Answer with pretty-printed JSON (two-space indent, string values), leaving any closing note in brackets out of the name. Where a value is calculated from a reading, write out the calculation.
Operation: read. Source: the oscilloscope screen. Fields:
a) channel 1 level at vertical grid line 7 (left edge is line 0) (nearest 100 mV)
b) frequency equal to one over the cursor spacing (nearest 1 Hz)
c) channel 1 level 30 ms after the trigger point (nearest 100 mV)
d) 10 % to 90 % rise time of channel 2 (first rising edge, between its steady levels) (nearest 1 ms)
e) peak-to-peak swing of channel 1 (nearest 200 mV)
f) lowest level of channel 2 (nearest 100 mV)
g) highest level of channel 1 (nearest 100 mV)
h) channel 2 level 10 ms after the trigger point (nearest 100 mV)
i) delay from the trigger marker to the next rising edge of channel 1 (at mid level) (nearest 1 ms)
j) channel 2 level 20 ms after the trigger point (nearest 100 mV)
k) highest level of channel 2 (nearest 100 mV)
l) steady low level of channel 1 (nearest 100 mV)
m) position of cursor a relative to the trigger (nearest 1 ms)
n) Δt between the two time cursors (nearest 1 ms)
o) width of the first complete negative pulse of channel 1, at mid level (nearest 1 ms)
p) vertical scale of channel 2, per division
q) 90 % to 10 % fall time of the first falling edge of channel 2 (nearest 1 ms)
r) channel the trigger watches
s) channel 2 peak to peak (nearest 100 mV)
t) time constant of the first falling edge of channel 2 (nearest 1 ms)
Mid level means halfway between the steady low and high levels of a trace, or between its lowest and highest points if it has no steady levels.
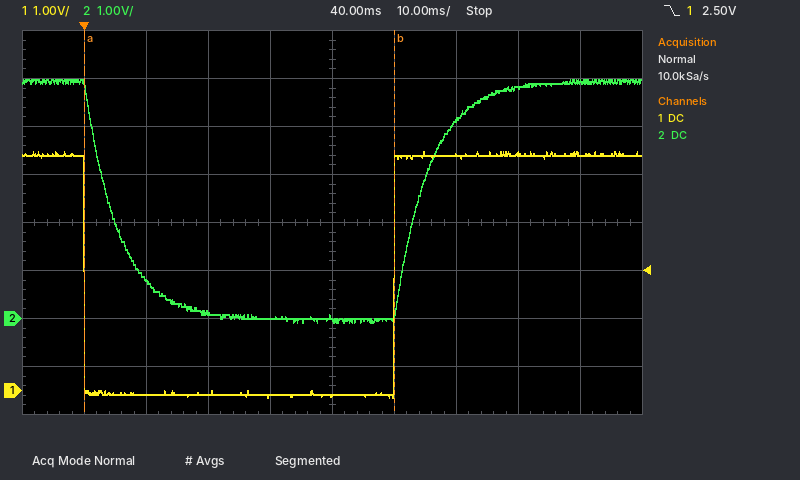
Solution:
{
  "channel 1 level at vertical grid line 7 (left edge is line 0)": "4.9 V",
  "frequency equal to one over the cursor spacing": "1 / 50 ms ≈ 20 Hz",
  "channel 1 level 30 ms after the trigger point": "-100 mV",
  "10 % to 90 % rise time of channel 2 (first rising edge, between its steady levels)": "12 ms",
  "peak-to-peak swing of channel 1": "5.2 V",
  "lowest level of channel 2": "-100 mV",
  "highest level of channel 1": "5.0 V",
  "channel 2 level 10 ms after the trigger point": "800 mV",
  "delay from the trigger marker to the next rising edge of channel 1 (at mid level)": "50 ms",
  "channel 2 level 20 ms after the trigger point": "100 mV",
  "highest level of channel 2": "5.0 V",
  "steady low level of channel 1": "-100 mV",
  "position of cursor a relative to the trigger": "0 ms",
  "Δt between the two time cursors": "50 ms",
  "width of the first complete negative pulse of channel 1, at mid level": "50 ms",
  "vertical scale of channel 2, per division": "1 V",
  "90 % to 10 % fall time of the first falling edge of channel 2": "12 ms",
  "channel the trigger watches": "channel 1",
  "channel 2 peak to peak": "5.0 V − (-100 mV) = 5.1 V",
  "time constant of the first falling edge of channel 2": "12 ms / 2.2 ≈ 5 ms"
}
